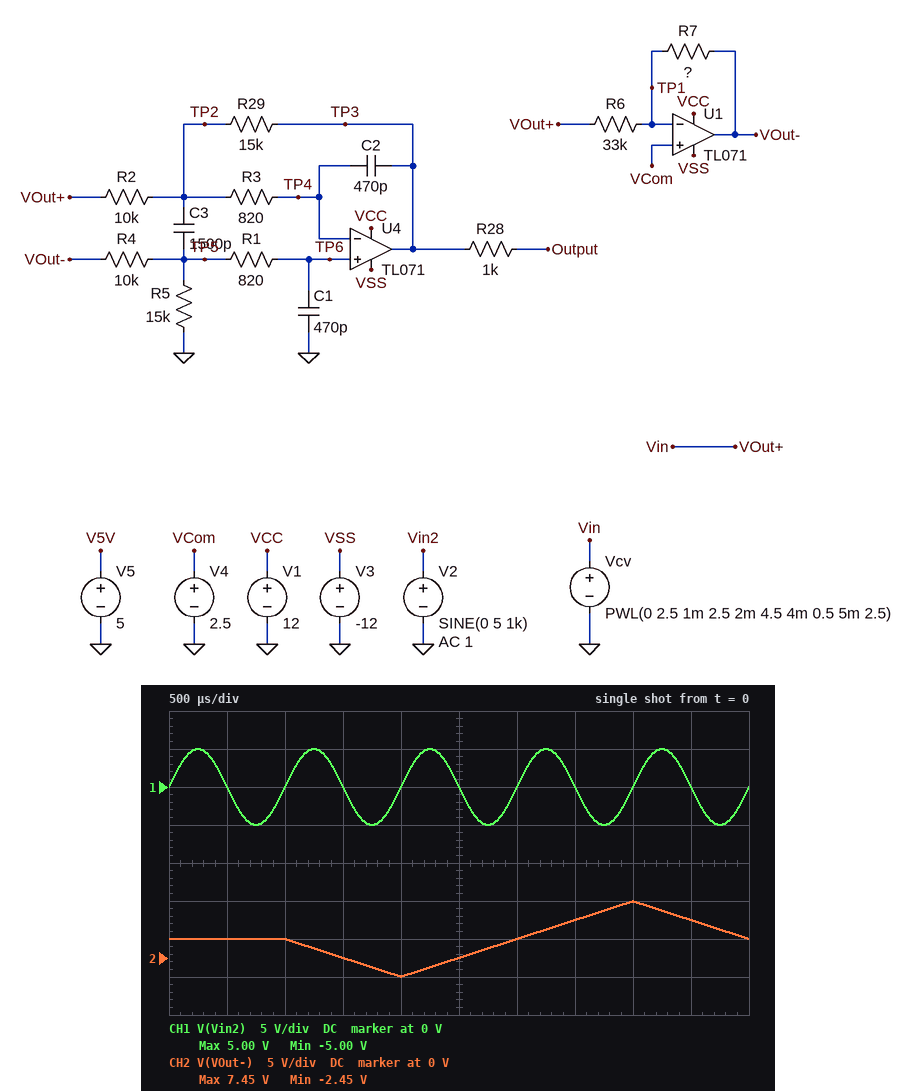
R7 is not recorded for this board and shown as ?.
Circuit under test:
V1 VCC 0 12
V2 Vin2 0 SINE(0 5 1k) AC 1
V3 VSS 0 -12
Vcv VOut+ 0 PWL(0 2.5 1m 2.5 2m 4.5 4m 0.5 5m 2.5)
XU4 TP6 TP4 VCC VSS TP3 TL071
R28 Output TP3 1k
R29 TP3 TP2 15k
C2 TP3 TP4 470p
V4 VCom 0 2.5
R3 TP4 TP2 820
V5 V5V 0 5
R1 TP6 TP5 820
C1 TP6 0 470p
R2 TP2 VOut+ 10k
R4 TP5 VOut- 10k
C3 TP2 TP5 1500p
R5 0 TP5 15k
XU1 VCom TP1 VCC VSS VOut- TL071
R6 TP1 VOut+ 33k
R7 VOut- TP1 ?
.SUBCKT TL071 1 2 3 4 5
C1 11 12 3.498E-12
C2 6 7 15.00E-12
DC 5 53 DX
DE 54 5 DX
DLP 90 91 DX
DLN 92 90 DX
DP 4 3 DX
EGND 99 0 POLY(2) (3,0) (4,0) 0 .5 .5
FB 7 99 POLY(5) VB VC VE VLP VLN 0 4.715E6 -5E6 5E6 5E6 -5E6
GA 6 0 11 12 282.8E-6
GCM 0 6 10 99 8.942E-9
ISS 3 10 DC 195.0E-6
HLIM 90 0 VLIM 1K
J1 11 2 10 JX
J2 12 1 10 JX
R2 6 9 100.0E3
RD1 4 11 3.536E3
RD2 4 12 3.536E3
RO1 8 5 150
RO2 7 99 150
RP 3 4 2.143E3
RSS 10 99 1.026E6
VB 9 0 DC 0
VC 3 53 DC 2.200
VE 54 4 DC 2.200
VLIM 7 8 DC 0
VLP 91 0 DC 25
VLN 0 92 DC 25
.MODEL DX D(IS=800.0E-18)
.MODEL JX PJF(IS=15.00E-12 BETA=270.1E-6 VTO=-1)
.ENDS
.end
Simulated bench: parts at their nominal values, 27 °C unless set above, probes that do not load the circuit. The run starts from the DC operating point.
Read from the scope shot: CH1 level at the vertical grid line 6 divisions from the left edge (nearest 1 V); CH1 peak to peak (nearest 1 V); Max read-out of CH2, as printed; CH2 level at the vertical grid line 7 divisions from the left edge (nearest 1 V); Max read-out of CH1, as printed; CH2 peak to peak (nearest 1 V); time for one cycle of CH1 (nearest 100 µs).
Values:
0 V
10 V
7.45 V
5 V
5.00 V
10 V
1.0 ms
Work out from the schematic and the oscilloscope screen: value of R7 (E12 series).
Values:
82 kΩ
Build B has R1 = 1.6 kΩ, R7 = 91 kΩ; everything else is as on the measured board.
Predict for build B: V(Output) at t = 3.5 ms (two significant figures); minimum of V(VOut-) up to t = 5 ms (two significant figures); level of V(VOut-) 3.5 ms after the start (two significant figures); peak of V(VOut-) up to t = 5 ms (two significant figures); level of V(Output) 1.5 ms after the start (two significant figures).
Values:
5.5 V
-3.0 V
5.3 V
8.0 V
-5.5 V
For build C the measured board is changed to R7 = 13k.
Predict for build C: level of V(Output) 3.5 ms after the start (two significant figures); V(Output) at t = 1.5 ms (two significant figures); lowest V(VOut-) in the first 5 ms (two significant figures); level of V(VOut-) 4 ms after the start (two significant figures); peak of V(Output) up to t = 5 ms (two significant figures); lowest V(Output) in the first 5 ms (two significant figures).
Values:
2.1 V
-2.1 V
1.7 V
3.3 V
4.2 V
-4.2 V
